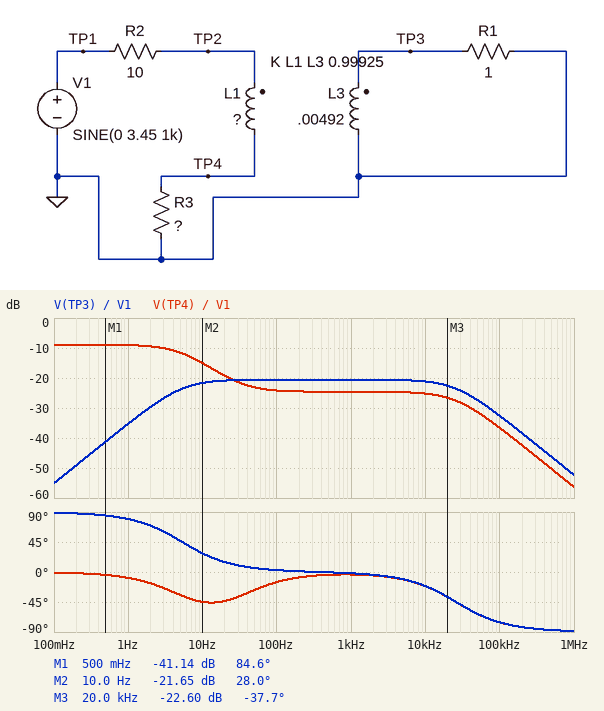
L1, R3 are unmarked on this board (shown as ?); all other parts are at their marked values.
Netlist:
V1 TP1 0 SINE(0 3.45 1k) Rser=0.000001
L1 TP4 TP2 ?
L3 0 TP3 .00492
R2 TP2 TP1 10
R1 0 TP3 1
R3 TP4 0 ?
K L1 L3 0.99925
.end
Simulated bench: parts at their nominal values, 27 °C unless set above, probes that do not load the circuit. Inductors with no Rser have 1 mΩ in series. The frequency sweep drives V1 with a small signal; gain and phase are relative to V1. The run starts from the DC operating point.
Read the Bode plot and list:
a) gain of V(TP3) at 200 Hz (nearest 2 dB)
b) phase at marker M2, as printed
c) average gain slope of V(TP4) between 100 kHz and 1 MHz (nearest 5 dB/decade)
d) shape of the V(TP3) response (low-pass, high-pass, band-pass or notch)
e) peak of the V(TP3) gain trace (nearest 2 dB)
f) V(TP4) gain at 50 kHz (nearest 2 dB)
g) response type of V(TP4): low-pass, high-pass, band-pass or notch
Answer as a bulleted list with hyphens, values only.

- -20 dB
- 28.0 deg
- -20 dB/decade
- band-pass
- -20 dB
- -32 dB
- low-pass
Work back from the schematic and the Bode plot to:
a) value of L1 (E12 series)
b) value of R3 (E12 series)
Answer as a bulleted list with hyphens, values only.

- 390 mH
- 5.6 Ω
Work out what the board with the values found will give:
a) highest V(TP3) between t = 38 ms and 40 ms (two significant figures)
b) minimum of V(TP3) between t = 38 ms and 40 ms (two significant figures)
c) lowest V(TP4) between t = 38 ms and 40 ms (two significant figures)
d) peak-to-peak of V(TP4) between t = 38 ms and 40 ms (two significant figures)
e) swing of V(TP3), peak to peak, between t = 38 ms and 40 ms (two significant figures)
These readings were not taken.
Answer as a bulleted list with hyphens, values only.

- 320 mV
- -320 mV
- -200 mV
- 410 mV
- 650 mV
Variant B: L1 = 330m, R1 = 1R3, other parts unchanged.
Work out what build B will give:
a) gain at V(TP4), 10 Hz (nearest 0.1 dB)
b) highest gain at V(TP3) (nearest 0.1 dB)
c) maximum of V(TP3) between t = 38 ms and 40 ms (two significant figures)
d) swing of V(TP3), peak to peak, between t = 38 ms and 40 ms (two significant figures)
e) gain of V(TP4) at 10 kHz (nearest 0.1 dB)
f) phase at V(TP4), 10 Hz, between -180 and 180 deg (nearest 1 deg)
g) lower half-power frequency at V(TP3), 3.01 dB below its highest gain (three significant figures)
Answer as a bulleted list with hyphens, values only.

- -14.0 dB
- -19.7 dB
- 360 mV
- 710 mV
- -25.7 dB
- -44 deg
- 6.38 Hz
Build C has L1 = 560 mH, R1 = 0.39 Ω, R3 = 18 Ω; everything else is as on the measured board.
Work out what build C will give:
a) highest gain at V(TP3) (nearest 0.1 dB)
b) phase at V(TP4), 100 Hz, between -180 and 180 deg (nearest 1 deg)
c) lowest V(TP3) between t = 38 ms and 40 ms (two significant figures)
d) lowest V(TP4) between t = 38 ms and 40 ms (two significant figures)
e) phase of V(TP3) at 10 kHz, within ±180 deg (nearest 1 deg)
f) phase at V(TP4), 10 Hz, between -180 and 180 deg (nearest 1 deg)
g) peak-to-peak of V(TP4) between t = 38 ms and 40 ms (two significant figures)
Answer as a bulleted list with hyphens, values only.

- -24.8 dB
- -5 deg
- -200 mV
- -850 mV
- -36 deg
- -26 deg
- 1.7 V
